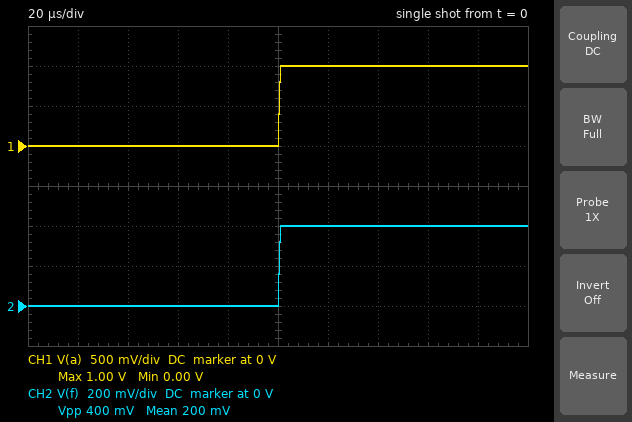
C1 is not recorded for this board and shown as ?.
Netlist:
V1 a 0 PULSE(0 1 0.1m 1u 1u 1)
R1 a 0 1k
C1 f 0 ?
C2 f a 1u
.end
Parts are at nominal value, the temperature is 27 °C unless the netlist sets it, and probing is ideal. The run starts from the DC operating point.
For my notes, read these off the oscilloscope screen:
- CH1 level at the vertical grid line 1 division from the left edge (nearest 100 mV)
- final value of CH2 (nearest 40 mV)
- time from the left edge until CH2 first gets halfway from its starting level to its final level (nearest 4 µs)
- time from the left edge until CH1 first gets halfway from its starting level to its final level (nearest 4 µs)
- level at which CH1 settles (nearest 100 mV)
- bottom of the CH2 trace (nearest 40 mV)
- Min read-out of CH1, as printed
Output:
0 V
400 mV
100 µs
100 µs
1.0 V
0 V
0.00 V
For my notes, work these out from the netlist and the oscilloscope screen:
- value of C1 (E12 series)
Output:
1.5 µF
